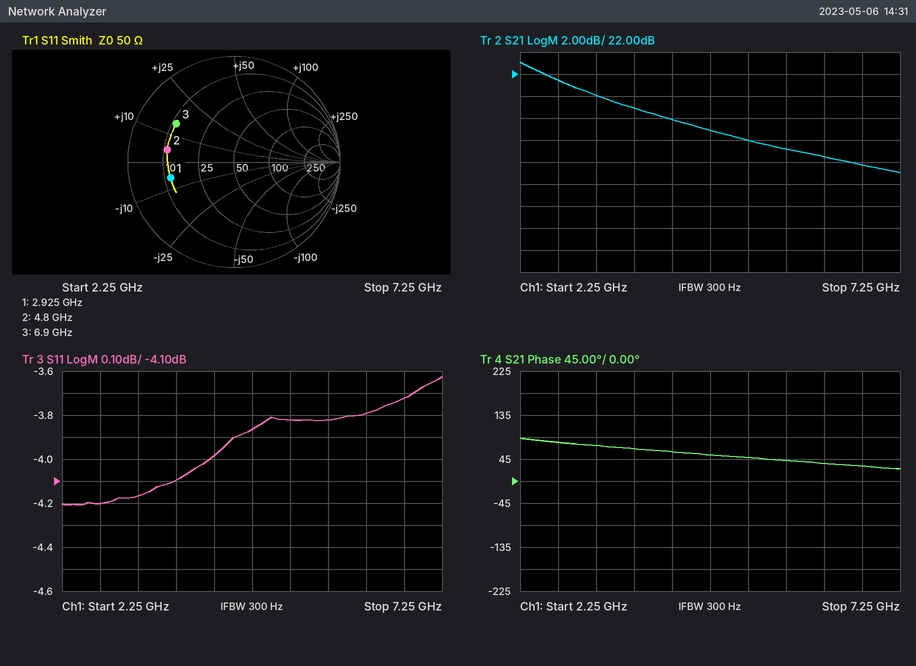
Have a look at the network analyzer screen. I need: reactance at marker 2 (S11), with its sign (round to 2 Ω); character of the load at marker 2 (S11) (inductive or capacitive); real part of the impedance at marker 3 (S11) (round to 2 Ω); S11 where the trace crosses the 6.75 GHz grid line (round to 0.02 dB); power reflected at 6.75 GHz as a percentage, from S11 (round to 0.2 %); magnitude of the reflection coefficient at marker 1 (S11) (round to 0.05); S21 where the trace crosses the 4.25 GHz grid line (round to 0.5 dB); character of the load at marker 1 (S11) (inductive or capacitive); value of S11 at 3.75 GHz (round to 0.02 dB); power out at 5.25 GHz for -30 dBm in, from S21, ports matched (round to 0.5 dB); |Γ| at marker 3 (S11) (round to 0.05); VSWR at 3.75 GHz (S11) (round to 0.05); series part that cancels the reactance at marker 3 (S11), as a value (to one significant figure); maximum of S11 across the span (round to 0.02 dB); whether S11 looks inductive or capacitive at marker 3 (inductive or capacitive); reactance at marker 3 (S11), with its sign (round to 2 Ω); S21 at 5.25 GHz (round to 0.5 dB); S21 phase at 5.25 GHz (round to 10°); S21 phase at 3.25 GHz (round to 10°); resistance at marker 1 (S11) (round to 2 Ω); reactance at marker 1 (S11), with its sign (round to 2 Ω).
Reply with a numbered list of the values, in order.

1. +4 Ω
2. inductive
3. 12 Ω
4. -3.72 dB
5. 42.4 %
6. 0.60
7. 18.0 dB
8. capacitive
9. -4.10 dB
10. -14.0 dBm
11. 0.65
12. 4.30
13. 2 pF
14. -3.62 dB
15. inductive
16. +14 Ω
17. 16.0 dB
18. 50°
19. 70°
20. 12 Ω
21. -6 Ω
